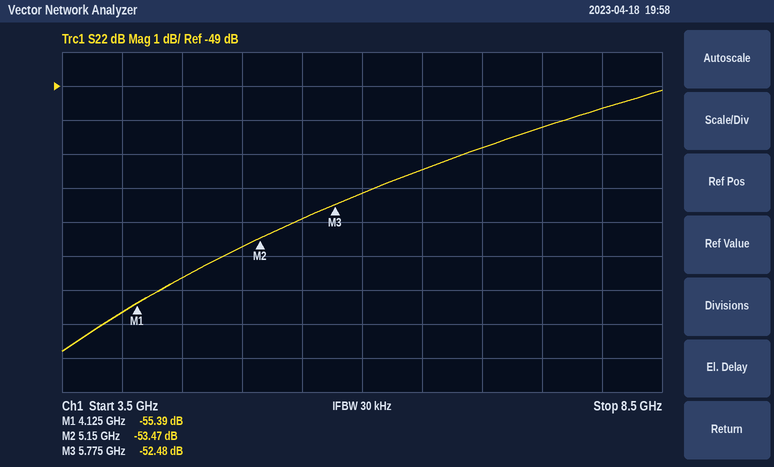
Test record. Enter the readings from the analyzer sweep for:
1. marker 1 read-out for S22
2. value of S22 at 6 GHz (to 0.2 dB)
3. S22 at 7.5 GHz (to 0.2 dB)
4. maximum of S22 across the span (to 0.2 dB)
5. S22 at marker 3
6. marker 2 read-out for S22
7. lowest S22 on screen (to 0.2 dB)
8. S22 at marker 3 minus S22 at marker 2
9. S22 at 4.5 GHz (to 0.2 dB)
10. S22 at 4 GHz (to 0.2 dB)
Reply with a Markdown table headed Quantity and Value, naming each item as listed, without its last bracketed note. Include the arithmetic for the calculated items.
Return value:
| Quantity | Value |
|---|---|
| marker 1 read-out for S22 | -55.39 dB |
| value of S22 at 6 GHz | -52.2 dB |
| S22 at 7.5 GHz | -50.2 dB |
| maximum of S22 across the span | -49.2 dB |
| S22 at marker 3 | -52.48 dB |
| marker 2 read-out for S22 | -53.47 dB |
| lowest S22 on screen | -56.8 dB |
| S22 at marker 3 minus S22 at marker 2 | -52.48 − (-53.47) = 0.99 dB |
| S22 at 4.5 GHz | -54.6 dB |
| S22 at 4 GHz | -55.6 dB |
